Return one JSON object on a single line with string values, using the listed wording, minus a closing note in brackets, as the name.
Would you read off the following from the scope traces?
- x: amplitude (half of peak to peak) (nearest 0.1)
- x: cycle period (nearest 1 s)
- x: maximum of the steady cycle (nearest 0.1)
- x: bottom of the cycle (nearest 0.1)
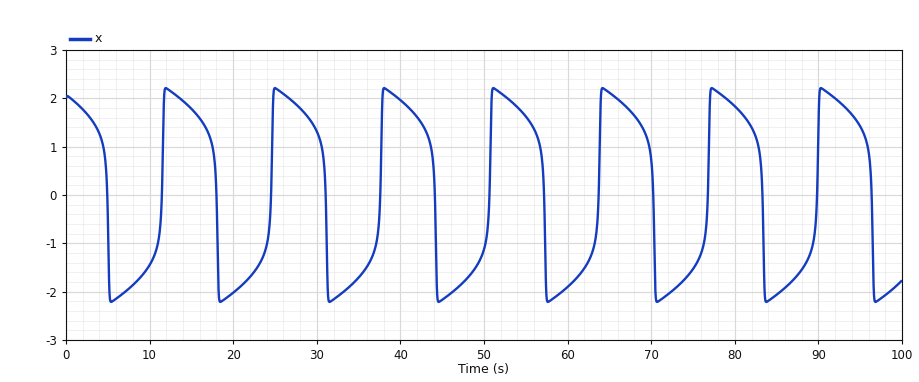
{"x: amplitude (half of peak to peak)": "2.2", "x: cycle period": "13 s", "x: maximum of the steady cycle": "2.2", "x: bottom of the cycle": "-2.2"}
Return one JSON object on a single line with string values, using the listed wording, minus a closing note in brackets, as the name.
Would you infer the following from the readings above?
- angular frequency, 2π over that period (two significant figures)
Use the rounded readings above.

{"angular frequency, 2π over that period": "0.48 rad/s"}
